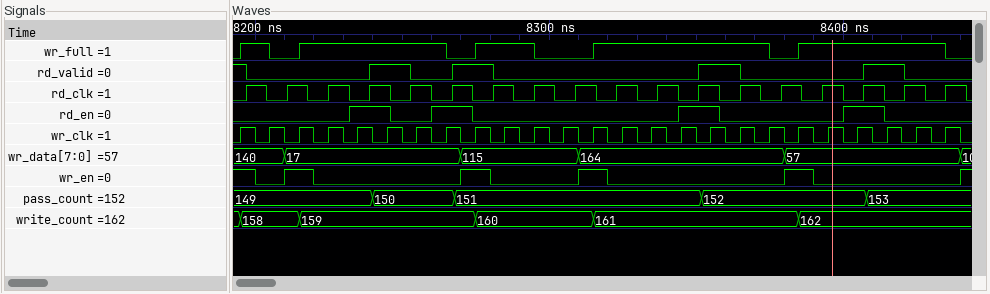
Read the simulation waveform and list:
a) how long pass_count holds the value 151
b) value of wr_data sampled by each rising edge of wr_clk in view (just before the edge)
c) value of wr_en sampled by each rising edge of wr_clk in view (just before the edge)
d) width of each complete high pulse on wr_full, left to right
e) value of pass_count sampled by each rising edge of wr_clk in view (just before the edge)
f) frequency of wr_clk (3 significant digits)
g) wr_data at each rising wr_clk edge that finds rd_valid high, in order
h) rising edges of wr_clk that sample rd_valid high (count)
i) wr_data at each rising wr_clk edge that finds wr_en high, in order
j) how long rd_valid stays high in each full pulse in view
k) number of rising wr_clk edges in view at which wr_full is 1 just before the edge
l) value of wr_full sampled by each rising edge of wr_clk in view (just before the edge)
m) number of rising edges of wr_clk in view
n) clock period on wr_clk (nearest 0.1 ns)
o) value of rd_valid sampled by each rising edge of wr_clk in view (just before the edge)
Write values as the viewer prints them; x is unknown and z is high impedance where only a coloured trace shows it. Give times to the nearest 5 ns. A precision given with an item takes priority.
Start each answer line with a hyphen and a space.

- 85 ns
- 140, 140, 17, 17, 17, 17, 17, 17, 115, 115, 115, 115, 164, 164, 164, 164, 164, 164, 164, 57, 57, 57, 57, 57, 57
- 1 0 1 0 0 0 0 0 1 0 0 0 1 0 0 0 0 0 0 1 0 0 0 0 0
- 10 ns, 50 ns, 20 ns, 60 ns, 50 ns
- 149, 149, 149, 149, 149, 150, 150, 150, 151, 151, 151, 151, 151, 151, 151, 151, 152, 152, 152, 152, 152, 152, 153, 153, 153
- 100 MHz
- 140, 17, 115, 164, 164, 57
- 6
- 140, 17, 115, 164, 57
- 15 ns, 15 ns, 15 ns, 15 ns
- 19
- 0 1 0 1 1 1 1 1 0 1 1 0 0 1 1 1 1 1 1 0 1 1 1 1 1
- 25
- 10 ns
- 1 0 0 0 0 1 0 0 1 0 0 0 0 0 0 0 1 1 0 0 0 0 1 0 0
